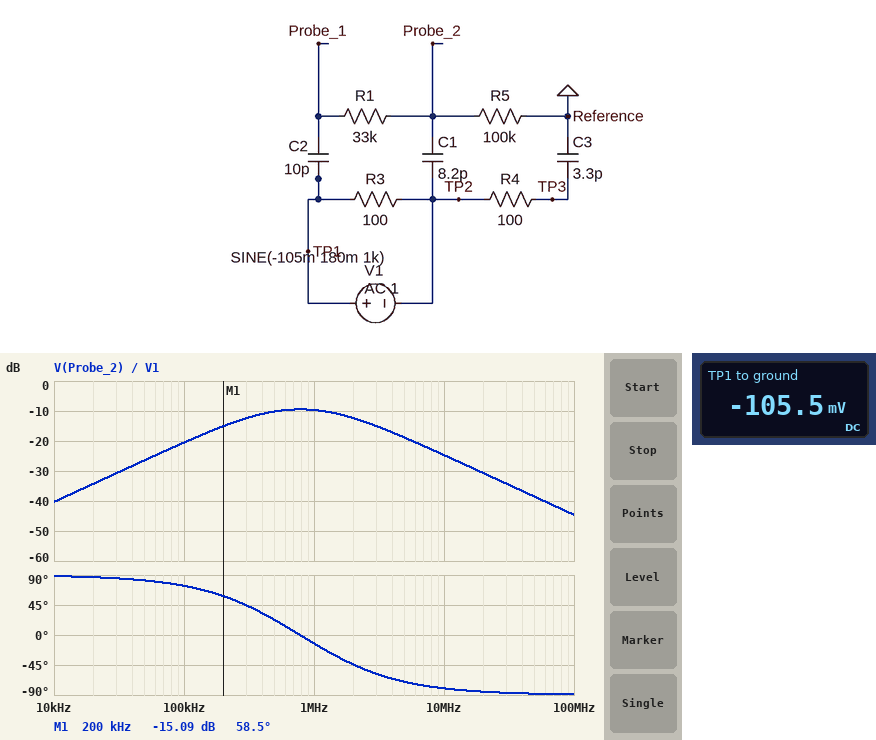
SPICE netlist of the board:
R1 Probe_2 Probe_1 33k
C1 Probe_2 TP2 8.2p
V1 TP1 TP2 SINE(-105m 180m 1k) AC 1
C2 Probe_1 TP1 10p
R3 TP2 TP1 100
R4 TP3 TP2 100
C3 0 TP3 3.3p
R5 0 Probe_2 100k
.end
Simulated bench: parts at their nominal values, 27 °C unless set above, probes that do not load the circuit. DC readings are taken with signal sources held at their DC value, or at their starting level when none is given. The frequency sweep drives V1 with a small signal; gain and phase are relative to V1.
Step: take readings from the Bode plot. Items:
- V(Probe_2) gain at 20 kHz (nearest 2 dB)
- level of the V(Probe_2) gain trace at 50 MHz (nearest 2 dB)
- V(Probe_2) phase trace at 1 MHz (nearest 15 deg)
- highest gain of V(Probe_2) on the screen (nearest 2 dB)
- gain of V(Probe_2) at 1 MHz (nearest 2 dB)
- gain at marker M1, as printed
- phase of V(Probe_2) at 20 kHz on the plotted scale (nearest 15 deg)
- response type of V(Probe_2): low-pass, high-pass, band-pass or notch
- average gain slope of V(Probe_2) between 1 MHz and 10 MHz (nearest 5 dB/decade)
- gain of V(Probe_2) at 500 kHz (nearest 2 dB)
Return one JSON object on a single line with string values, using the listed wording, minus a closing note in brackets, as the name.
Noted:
{"V(Probe_2) gain at 20 kHz": "-34 dB", "level of the V(Probe_2) gain trace at 50 MHz": "-38 dB", "V(Probe_2) phase trace at 1 MHz": "-15 deg", "highest gain of V(Probe_2) on the screen": "-10 dB", "gain of V(Probe_2) at 1 MHz": "-10 dB", "gain at marker M1, as printed": "-15.09 dB", "phase of V(Probe_2) at 20 kHz on the plotted scale": "90 deg", "response type of V(Probe_2): low-pass, high-pass, band-pass or notch": "band-pass", "average gain slope of V(Probe_2) between 1 MHz and 10 MHz": "-15 dB/decade", "gain of V(Probe_2) at 500 kHz": "-10 dB"}
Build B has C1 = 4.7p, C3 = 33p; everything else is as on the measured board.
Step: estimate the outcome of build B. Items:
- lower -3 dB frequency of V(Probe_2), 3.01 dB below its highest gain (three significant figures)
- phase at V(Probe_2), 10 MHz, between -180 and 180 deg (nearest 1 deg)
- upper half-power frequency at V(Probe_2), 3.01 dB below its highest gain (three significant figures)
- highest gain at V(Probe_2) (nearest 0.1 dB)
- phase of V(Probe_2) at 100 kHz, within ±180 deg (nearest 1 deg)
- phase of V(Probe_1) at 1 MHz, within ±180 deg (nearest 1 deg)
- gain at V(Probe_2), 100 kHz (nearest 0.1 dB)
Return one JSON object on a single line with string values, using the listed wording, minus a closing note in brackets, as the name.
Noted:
{"lower -3 dB frequency of V(Probe_2), 3.01 dB below its highest gain": "117 kHz", "phase at V(Probe_2), 10 MHz, between -180 and 180 deg": "-79 deg", "upper half-power frequency at V(Probe_2), 3.01 dB below its highest gain": "2.01 MHz", "highest gain at V(Probe_2)": "-5.3 dB", "phase of V(Probe_2) at 100 kHz, within ±180 deg": "50 deg", "phase of V(Probe_1) at 1 MHz, within ±180 deg": "13 deg", "gain at V(Probe_2), 100 kHz": "-9.2 dB"}
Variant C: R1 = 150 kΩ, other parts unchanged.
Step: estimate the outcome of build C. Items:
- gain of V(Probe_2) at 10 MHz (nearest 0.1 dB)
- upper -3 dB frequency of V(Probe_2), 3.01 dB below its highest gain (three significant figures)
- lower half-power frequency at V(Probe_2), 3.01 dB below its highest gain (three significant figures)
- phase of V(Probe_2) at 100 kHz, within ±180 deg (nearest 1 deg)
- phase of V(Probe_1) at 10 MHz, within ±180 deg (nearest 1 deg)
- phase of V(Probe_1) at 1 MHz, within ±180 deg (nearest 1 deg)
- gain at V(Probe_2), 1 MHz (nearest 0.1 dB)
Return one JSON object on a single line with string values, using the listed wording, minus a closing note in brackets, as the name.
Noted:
{"gain of V(Probe_2) at 10 MHz": "-37.8 dB", "upper -3 dB frequency of V(Probe_2), 3.01 dB below its highest gain": "1.04 MHz", "lower half-power frequency at V(Probe_2), 3.01 dB below its highest gain": "129 kHz", "phase of V(Probe_2) at 100 kHz, within ±180 deg": "54 deg", "phase of V(Probe_1) at 10 MHz, within ±180 deg": "1 deg", "phase of V(Probe_1) at 1 MHz, within ±180 deg": "8 deg", "gain at V(Probe_2), 1 MHz": "-19.8 dB"}
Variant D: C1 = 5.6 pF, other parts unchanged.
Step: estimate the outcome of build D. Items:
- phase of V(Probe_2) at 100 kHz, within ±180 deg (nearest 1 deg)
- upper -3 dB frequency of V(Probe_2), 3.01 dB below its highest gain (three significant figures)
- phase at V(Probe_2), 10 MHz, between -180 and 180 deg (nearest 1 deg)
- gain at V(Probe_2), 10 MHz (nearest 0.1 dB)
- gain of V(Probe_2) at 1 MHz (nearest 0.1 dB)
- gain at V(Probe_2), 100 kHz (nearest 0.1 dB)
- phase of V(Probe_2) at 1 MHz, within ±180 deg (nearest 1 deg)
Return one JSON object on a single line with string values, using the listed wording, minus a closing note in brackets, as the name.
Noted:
{"phase of V(Probe_2) at 100 kHz, within ±180 deg": "75 deg", "upper -3 dB frequency of V(Probe_2), 3.01 dB below its highest gain": "2.43 MHz", "phase at V(Probe_2), 10 MHz, between -180 and 180 deg": "-78 deg", "gain at V(Probe_2), 10 MHz": "-21.4 dB", "gain of V(Probe_2) at 1 MHz": "-7.8 dB", "gain at V(Probe_2), 100 kHz": "-19.4 dB", "phase of V(Probe_2) at 1 MHz, within ±180 deg": "-6 deg"}
